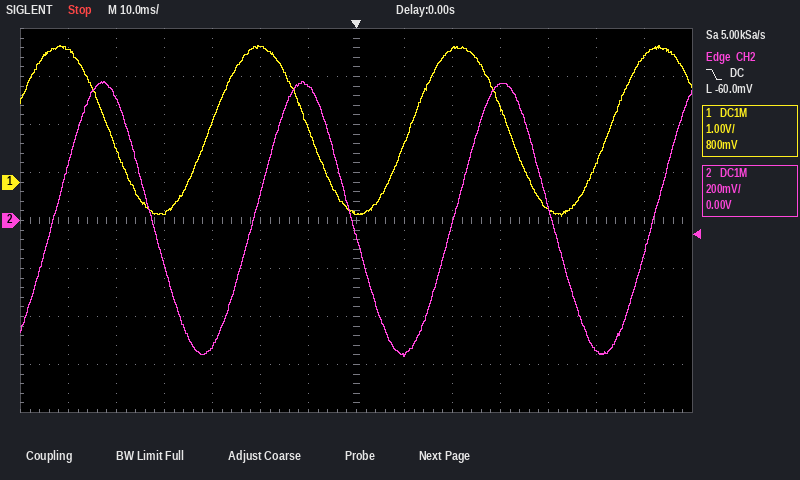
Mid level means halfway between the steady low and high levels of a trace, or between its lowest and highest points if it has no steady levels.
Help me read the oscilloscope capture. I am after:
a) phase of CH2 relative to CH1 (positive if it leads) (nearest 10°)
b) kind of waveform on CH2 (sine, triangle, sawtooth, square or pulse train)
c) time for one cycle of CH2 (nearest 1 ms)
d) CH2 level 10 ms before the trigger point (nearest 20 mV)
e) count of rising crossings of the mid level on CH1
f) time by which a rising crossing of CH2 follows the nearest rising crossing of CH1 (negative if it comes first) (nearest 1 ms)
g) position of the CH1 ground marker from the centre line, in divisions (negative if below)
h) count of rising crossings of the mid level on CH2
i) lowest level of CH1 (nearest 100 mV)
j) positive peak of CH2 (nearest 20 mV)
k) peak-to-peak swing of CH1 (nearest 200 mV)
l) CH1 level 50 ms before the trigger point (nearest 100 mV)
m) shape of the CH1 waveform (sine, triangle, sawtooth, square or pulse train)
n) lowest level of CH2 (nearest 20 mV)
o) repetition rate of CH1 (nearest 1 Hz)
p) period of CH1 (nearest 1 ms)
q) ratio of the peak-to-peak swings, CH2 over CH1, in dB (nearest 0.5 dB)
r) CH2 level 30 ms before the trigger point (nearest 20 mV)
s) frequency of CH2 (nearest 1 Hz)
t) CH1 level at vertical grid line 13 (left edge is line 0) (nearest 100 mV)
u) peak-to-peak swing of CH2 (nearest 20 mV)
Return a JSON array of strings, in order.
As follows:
["-80°", "sine", "42 ms", "560 mV", "3", "+9 ms", "+0.8 div", "4", "-700 mV", "580 mV", "3.6 V", "700 mV", "sine", "-560 mV", "24 Hz", "42 ms", "-10.0 dB", "-520 mV", "24 Hz", "2.6 V", "1.14 V"]
